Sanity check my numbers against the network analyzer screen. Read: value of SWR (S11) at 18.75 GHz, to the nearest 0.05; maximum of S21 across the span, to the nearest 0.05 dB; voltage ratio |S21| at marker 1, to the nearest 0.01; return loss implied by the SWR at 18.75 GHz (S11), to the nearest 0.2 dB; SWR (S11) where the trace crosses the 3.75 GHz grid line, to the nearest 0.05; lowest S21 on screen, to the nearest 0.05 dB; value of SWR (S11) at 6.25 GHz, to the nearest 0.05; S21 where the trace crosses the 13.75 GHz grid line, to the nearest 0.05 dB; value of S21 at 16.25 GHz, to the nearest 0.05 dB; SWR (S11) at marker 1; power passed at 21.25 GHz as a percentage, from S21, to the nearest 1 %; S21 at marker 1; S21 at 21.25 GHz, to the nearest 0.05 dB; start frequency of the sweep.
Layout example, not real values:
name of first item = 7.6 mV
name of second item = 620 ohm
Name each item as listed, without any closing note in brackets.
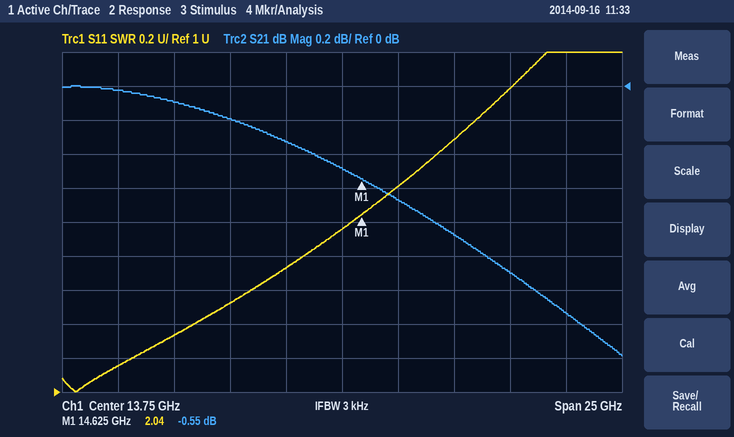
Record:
value of SWR (S11) at 18.75 GHz, to the nearest 0.05 = 2.50
maximum of S21 across the span, to the nearest 0.05 dB = 0.00 dB
voltage ratio |S21| at marker 1, to the nearest 0.01 = 0.94
return loss implied by the SWR at 18.75 GHz (S11), to the nearest 0.2 dB = 7.4 dB
SWR (S11) where the trace crosses the 3.75 GHz grid line, to the nearest 0.05 = 1.15
lowest S21 on screen, to the nearest 0.05 dB = -1.60 dB
value of SWR (S11) at 6.25 GHz, to the nearest 0.05 = 1.35
S21 where the trace crosses the 13.75 GHz grid line, to the nearest 0.05 dB = -0.50 dB
value of S21 at 16.25 GHz, to the nearest 0.05 dB = -0.65 dB
SWR (S11) at marker 1 = 2.04
power passed at 21.25 GHz as a percentage, from S21, to the nearest 1 % = 78 %
S21 at marker 1 = -0.55 dB
S21 at 21.25 GHz, to the nearest 0.05 dB = -1.10 dB
start frequency of the sweep = 1.25 GHz
